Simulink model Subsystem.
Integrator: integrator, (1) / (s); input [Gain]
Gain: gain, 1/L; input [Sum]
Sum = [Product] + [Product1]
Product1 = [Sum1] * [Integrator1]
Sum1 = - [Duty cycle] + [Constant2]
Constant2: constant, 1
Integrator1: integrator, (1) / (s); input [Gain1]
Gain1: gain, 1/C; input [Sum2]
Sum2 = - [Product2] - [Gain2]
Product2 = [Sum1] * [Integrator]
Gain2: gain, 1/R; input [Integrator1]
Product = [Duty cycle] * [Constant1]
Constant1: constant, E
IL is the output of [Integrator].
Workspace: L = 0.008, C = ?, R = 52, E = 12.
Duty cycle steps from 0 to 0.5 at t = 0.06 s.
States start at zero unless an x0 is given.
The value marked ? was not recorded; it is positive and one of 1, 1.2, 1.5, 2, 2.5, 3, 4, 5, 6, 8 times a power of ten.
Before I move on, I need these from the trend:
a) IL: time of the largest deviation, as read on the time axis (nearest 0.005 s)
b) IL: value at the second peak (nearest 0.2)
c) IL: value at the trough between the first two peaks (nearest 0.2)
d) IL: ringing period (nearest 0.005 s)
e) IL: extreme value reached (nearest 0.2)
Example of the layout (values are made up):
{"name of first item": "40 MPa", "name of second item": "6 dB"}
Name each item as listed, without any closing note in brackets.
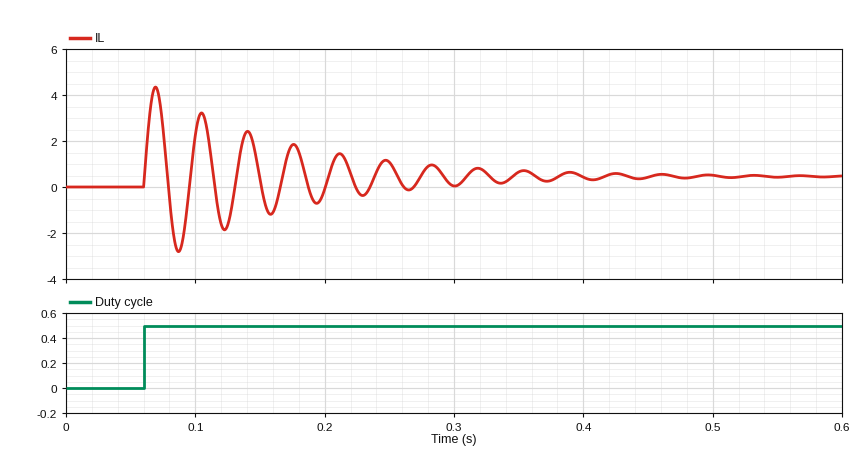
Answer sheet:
{"IL: time of the largest deviation, as read on the time axis": "0.070 s", "IL: value at the second peak": "3.2", "IL: value at the trough between the first two peaks": "-2.8", "IL: ringing period": "0.035 s", "IL: extreme value reached": "4.4"}
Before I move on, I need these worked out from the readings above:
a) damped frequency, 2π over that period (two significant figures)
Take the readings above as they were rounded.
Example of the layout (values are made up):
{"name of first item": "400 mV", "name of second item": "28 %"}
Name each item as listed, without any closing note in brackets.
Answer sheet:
{"damped frequency, 2π over that period": "180 rad/s"}
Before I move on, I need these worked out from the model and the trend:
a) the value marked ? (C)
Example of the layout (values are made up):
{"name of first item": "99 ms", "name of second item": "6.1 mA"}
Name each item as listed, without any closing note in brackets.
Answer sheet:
{"the value marked ?": "0.001"}
